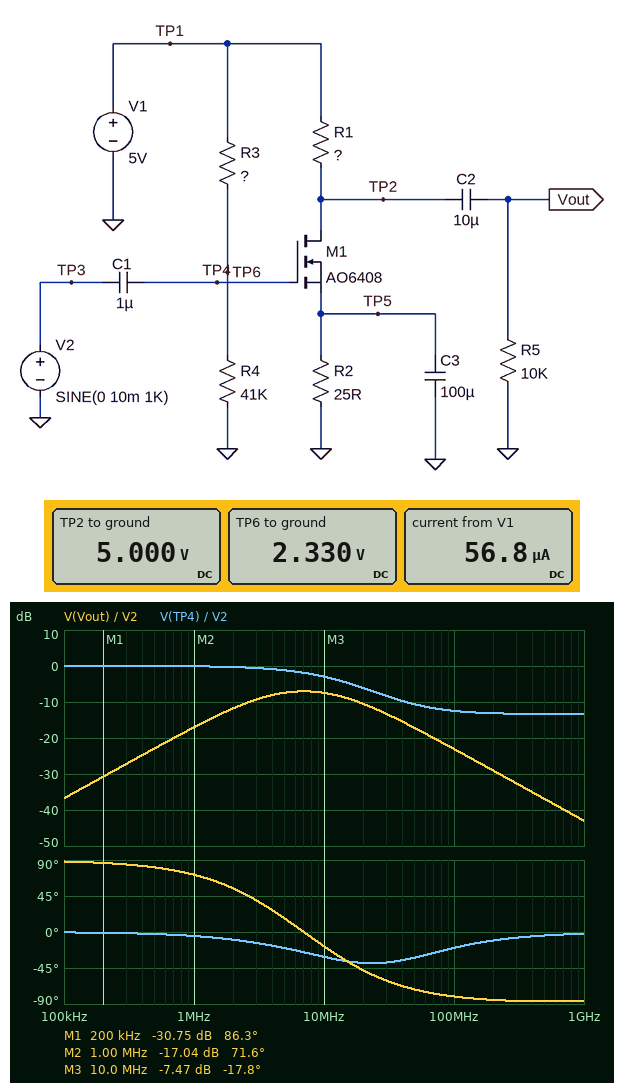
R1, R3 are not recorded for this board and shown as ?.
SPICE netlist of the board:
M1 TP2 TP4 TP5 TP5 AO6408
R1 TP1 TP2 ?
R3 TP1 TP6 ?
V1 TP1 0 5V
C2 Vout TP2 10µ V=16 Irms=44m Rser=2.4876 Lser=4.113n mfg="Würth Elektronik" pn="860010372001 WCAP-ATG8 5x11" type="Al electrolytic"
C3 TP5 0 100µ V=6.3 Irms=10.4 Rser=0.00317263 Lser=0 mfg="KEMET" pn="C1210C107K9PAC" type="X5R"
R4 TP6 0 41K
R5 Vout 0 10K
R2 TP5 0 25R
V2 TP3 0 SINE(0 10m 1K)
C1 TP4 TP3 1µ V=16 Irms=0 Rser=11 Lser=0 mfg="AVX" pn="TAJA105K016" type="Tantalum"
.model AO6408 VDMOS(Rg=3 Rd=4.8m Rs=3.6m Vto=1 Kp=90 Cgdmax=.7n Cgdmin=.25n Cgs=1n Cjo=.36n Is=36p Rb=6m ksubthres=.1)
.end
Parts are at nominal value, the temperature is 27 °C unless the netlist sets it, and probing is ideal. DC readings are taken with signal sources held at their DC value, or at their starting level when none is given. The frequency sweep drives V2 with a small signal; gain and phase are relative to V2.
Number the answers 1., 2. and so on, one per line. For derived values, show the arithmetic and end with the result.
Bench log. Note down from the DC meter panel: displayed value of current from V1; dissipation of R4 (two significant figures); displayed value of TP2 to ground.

1. 56.8 µA
2. (2.33 V)^2 / 41 kΩ = 130 µW
3. 5.000 V
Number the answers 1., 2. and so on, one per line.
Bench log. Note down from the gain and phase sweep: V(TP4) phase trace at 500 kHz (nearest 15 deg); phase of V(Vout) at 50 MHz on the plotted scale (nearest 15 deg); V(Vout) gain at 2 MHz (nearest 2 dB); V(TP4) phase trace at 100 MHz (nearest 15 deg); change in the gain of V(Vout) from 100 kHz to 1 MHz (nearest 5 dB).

1. 0 deg
2. -75 deg
3. -12 dB
4. -15 deg
5. 20 dB
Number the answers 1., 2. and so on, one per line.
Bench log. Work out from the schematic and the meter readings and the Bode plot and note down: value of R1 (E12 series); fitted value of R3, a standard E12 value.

1. 82 Ω
2. 47 kΩ
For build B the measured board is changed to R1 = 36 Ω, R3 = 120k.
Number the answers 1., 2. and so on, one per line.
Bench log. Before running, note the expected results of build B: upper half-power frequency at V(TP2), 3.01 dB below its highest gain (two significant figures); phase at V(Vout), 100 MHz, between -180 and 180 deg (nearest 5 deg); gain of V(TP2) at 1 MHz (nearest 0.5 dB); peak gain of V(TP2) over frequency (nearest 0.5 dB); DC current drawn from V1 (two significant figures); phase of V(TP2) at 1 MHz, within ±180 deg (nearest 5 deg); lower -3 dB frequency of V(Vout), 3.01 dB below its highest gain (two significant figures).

1. 27 MHz
2. -75 deg
3. -24.0 dB
4. -10.0 dB
5. 31 µA
6. 80 deg
7. 4.1 MHz
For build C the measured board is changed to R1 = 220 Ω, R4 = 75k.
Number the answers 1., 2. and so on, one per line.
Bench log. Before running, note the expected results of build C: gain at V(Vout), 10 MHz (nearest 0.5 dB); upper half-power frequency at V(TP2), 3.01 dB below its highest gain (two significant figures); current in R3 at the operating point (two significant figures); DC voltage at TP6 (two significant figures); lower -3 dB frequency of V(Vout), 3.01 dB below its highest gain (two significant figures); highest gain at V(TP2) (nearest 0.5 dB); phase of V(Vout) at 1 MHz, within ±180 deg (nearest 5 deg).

1. -6.5 dB
2. 14 MHz
3. 41 µA
4. 3.1 V
5. 1.3 MHz
6. -5.0 dB
7. 55 deg
